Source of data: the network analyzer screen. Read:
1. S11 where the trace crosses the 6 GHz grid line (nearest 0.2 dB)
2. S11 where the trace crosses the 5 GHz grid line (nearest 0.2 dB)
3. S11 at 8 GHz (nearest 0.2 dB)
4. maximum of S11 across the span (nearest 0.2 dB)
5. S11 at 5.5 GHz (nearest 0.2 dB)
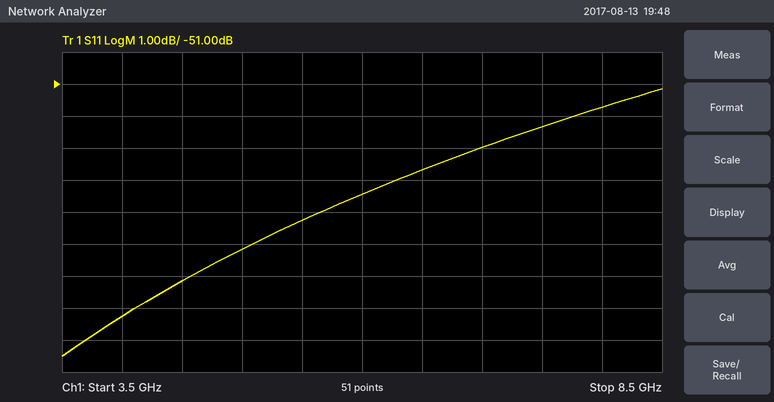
-54.4 dB
-56.2 dB
-51.8 dB
-51.2 dB
-55.2 dB
